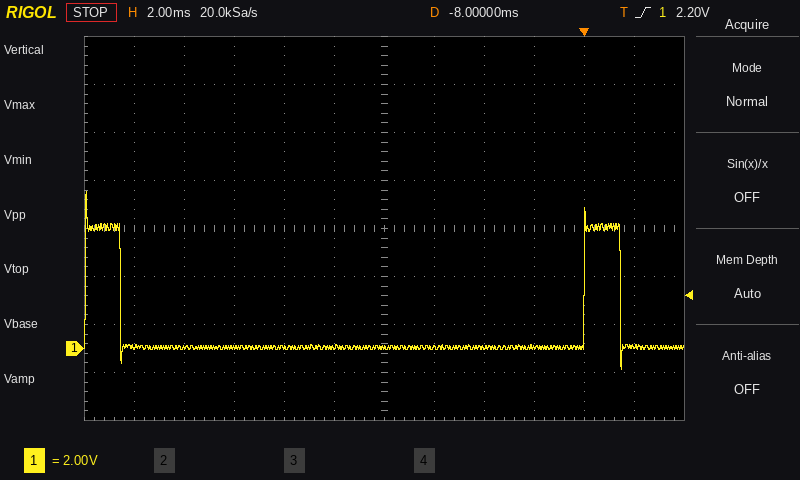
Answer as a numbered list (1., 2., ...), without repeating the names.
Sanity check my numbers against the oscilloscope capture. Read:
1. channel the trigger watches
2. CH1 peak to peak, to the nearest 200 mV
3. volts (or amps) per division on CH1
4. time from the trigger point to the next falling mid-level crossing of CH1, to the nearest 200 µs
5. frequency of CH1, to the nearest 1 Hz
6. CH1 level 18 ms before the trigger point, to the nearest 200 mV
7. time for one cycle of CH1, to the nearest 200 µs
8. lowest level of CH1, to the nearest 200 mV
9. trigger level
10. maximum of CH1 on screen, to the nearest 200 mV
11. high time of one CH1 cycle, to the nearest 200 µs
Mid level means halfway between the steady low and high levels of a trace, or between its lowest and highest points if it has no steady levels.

1. CH1
2. 7.4 V
3. 2 V
4. 1.4 ms
5. 50 Hz
6. 0.0 V
7. 20.0 ms
8. -800 mV
9. 2.20 V
10. 6.6 V
11. 1.4 ms
